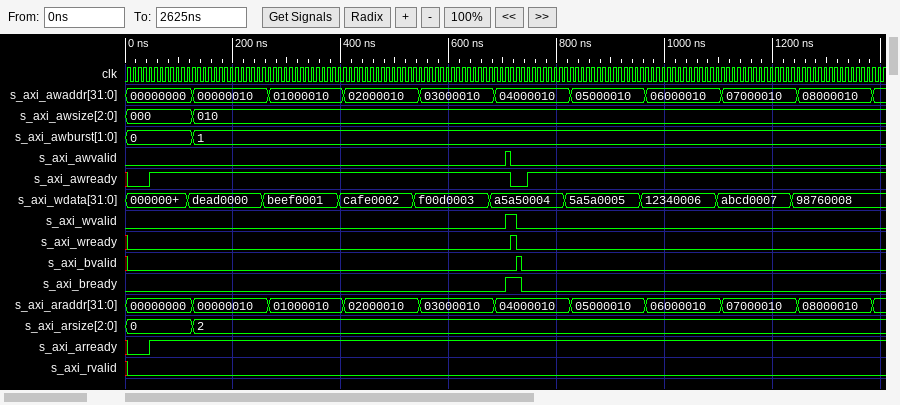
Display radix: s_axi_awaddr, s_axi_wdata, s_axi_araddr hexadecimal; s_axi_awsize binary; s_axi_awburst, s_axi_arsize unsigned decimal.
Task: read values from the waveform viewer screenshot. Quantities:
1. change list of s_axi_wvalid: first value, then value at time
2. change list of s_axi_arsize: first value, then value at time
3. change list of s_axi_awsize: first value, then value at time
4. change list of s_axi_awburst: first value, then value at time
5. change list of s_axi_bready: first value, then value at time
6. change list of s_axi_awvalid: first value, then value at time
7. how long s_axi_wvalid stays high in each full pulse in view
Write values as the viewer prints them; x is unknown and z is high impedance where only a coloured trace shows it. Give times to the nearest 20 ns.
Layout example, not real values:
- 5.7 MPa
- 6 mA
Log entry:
- 0, 1 at 700 ns, 0 at 720 ns
- 0, 2 at 120 ns
- 000, 010 at 120 ns
- 0, 1 at 120 ns
- 0, 1 at 700 ns, 0 at 740 ns
- 0, 1 at 700 ns, 0 at 720 ns
- 20 ns
